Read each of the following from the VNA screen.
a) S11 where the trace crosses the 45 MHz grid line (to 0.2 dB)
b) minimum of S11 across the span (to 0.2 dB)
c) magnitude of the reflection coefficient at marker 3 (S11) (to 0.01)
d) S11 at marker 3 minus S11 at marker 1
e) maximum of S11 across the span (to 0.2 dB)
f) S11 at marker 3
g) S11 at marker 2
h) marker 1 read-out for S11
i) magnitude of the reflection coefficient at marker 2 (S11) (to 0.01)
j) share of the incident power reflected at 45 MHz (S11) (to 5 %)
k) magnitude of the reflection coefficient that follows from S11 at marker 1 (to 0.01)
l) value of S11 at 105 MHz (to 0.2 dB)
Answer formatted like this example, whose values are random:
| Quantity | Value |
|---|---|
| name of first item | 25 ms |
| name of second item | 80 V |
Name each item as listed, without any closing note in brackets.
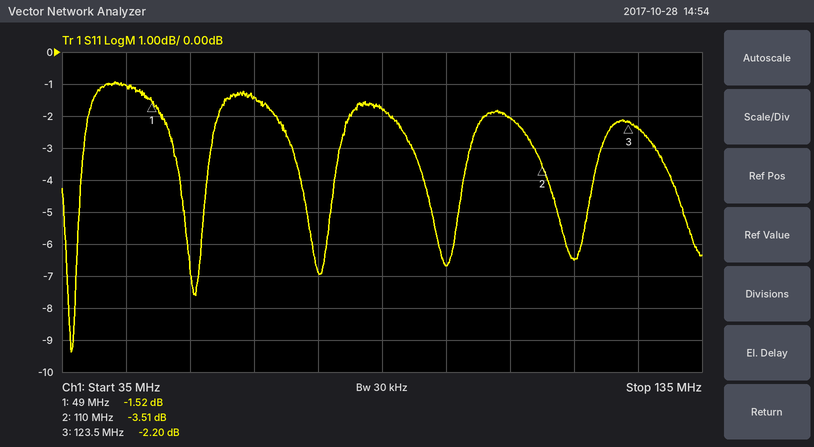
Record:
| Quantity | Value |
|---|---|
| S11 where the trace crosses the 45 MHz grid line | -1.0 dB |
| minimum of S11 across the span | -9.4 dB |
| magnitude of the reflection coefficient at marker 3 (S11) | 0.78 |
| S11 at marker 3 minus S11 at marker 1 | -0.68 dB |
| maximum of S11 across the span | -1.0 dB |
| S11 at marker 3 | -2.20 dB |
| S11 at marker 2 | -3.51 dB |
| marker 1 read-out for S11 | -1.52 dB |
| magnitude of the reflection coefficient at marker 2 (S11) | 0.67 |
| share of the incident power reflected at 45 MHz (S11) | 80 % |
| magnitude of the reflection coefficient that follows from S11 at marker 1 | 0.84 |
| value of S11 at 105 MHz | -2.0 dB |
